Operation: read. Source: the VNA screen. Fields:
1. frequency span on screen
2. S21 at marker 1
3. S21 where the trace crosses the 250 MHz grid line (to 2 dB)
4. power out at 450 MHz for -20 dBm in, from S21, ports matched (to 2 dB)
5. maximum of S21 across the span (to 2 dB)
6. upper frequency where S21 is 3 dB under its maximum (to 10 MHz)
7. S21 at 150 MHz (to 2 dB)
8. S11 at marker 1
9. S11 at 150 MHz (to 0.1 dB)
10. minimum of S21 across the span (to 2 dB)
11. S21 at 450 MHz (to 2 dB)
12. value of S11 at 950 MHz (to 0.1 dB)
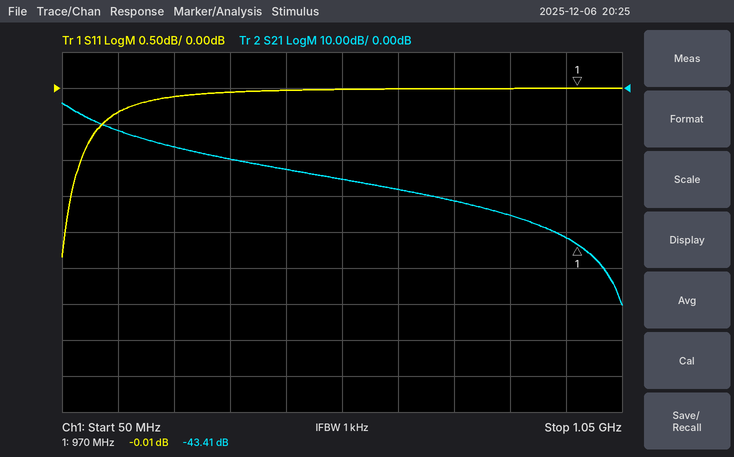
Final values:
1 GHz
-43.41 dB
-16 dB
-42 dBm
-4 dB
80 MHz
-12 dB
-0.01 dB
-0.3 dB
-60 dB
-22 dB
0.0 dB
